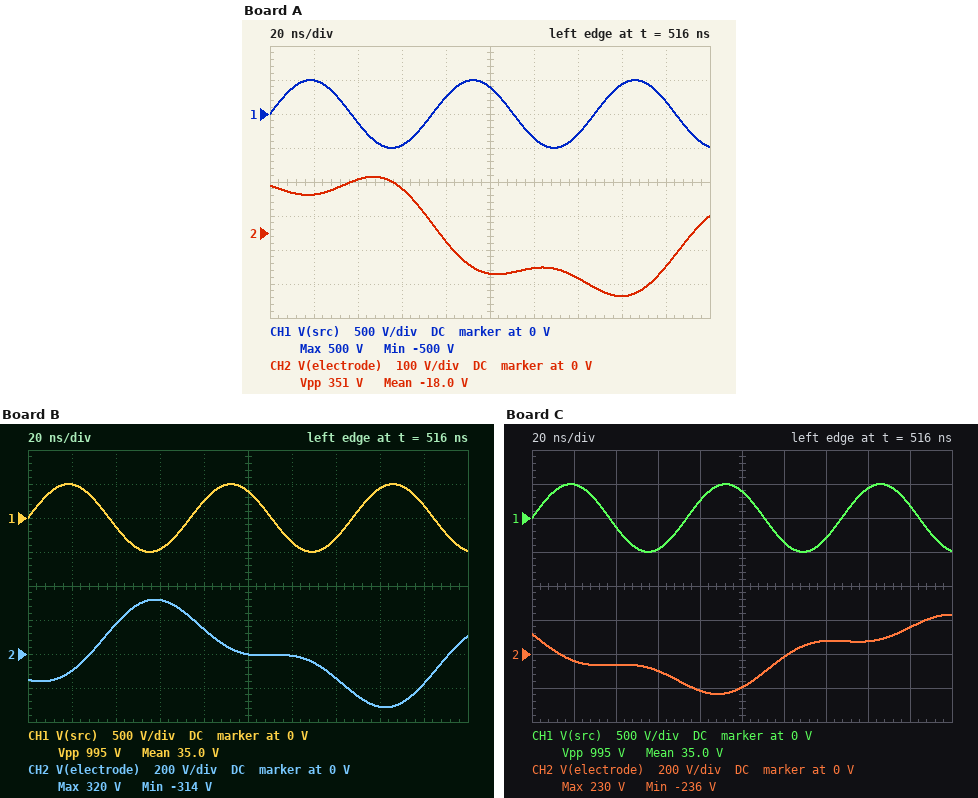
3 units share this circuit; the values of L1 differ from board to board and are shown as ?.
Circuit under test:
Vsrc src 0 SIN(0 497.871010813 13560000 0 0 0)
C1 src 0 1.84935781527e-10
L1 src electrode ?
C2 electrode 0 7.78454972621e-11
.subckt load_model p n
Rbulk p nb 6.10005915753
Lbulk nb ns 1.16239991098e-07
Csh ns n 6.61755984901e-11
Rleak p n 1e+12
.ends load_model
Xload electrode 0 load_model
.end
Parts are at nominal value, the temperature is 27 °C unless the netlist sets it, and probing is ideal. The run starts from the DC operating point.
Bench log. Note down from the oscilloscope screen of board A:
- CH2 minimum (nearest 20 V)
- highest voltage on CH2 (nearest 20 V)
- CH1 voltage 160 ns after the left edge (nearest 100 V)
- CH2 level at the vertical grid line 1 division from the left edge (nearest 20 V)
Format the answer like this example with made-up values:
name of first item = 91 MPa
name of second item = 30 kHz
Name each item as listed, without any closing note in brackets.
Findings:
CH2 minimum = -180 V
highest voltage on CH2 = 160 V
CH1 voltage 160 ns after the left edge = 400 V
CH2 level at the vertical grid line 1 division from the left edge = 120 V
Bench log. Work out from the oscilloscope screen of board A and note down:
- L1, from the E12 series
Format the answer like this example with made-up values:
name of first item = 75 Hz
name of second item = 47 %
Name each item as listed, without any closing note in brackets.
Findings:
L1, from the E12 series = 10 µH
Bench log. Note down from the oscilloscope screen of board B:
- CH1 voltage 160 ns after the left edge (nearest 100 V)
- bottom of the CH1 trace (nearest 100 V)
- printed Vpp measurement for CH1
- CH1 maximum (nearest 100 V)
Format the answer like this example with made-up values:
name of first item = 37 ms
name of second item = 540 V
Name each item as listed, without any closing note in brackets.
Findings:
CH1 voltage 160 ns after the left edge = 400 V
bottom of the CH1 trace = -500 V
printed Vpp measurement for CH1 = 995 V
CH1 maximum = 500 V
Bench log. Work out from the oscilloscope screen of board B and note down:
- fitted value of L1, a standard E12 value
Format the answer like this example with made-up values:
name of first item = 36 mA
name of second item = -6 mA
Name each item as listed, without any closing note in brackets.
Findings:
fitted value of L1, a standard E12 value = 5.6 µH
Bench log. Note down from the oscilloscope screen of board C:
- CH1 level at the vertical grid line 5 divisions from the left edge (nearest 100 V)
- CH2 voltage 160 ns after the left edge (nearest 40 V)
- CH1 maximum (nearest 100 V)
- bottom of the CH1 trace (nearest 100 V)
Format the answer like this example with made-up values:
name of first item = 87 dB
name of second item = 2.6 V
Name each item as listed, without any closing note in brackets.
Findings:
CH1 level at the vertical grid line 5 divisions from the left edge = 400 V
CH2 voltage 160 ns after the left edge = 80 V
CH1 maximum = 500 V
bottom of the CH1 trace = -500 V
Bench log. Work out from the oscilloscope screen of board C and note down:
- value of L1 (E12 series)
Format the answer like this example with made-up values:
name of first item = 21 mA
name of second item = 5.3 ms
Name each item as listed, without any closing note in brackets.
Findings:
value of L1 = 8.2 µH
